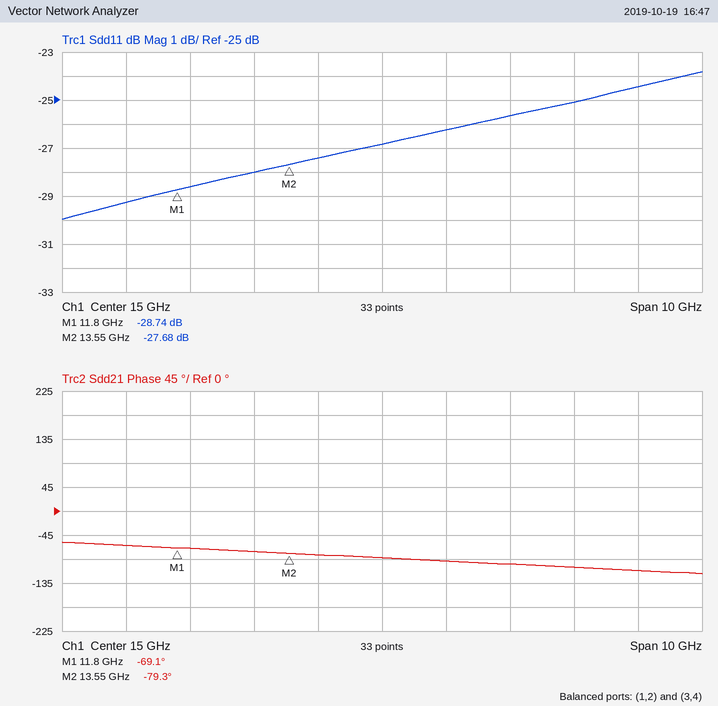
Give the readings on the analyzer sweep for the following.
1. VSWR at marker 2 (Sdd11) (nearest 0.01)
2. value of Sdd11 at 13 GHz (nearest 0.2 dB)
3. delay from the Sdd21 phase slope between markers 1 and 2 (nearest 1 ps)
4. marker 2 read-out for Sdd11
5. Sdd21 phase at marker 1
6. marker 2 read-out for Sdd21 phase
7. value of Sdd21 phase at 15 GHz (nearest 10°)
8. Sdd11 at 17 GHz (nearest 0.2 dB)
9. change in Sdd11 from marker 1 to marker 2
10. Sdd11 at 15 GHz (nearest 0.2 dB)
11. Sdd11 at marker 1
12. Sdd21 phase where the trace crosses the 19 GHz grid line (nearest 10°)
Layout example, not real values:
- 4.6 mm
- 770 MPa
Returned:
- 1.09
- -28.0 dB
- 16 ps
- -27.68 dB
- -69.1°
- -79.3°
- -90°
- -25.6 dB
- 1.06 dB
- -26.8 dB
- -28.74 dB
- -110°
